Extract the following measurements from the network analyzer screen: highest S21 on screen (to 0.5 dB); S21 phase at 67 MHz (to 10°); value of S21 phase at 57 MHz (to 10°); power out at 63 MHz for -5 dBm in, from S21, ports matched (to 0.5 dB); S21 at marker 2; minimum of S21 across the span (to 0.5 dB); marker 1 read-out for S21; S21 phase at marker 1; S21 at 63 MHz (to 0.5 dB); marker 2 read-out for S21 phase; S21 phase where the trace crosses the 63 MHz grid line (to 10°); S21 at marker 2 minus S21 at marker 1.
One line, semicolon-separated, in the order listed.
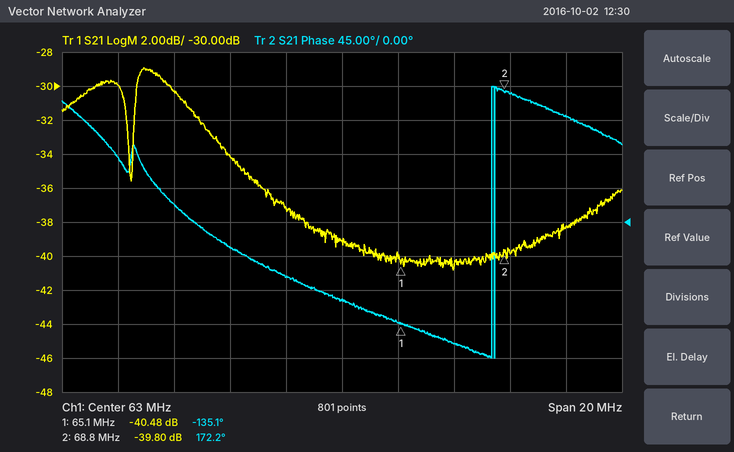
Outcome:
-29.0 dB; -160°; 20°; -44.0 dBm; -39.80 dB; -41.0 dB; -40.48 dB; -135.1°; -39.0 dB; 172.2°; -100°; 0.68 dB
